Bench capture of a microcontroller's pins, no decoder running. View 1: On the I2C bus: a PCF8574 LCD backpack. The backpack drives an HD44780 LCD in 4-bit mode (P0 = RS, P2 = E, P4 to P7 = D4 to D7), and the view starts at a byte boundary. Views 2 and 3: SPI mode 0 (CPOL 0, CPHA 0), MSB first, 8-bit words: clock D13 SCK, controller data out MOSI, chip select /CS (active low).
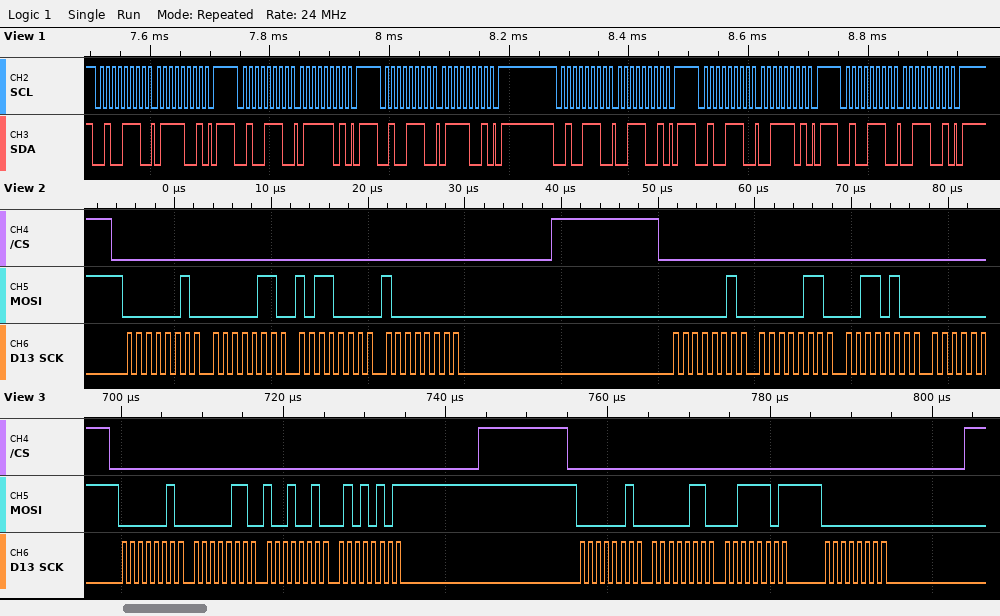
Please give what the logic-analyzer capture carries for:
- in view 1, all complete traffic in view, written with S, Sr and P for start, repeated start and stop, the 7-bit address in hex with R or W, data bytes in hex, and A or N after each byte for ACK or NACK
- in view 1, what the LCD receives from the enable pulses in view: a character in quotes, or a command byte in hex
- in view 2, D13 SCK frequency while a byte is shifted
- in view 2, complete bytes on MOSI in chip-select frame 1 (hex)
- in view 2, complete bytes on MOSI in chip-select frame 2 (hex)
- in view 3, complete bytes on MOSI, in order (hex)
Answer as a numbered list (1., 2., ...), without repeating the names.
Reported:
1. S 27W A 79 A P S 27W A 7D A P S 27W A 79 A P S 27W A 39 A P S 27W A 3D A P S 27W A 39 A P
2. 's'
3. 1 MHz
4. 02 06 B0 80
5. 02 06 34
6. 02 06 92 55 02 06 3D 00
